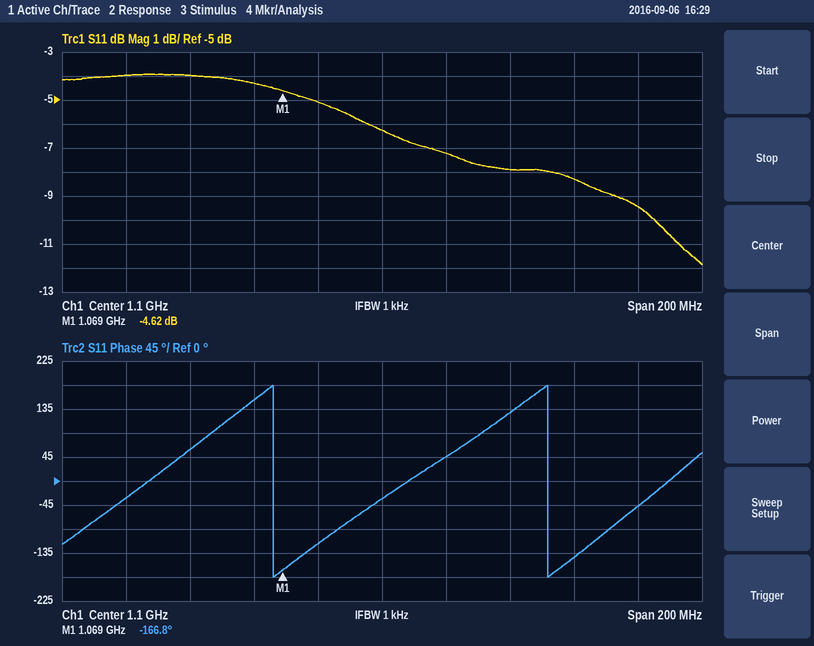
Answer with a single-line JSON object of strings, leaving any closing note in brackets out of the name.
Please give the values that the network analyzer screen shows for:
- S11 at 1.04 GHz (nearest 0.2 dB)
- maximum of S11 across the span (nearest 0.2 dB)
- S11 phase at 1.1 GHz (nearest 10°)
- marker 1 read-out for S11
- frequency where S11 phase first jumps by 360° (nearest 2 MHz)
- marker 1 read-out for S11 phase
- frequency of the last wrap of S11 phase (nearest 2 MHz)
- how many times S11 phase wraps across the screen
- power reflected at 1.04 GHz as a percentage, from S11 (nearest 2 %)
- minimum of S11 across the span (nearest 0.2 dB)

{"S11 at 1.04 GHz": "-4.0 dB", "maximum of S11 across the span": "-4.0 dB", "S11 phase at 1.1 GHz": "-30°", "marker 1 read-out for S11": "-4.62 dB", "frequency where S11 phase first jumps by 360°": "1.066 GHz", "marker 1 read-out for S11 phase": "-166.8°", "frequency of the last wrap of S11 phase": "1.152 GHz", "how many times S11 phase wraps across the screen": "2", "power reflected at 1.04 GHz as a percentage, from S11": "40 %", "minimum of S11 across the span": "-11.8 dB"}
